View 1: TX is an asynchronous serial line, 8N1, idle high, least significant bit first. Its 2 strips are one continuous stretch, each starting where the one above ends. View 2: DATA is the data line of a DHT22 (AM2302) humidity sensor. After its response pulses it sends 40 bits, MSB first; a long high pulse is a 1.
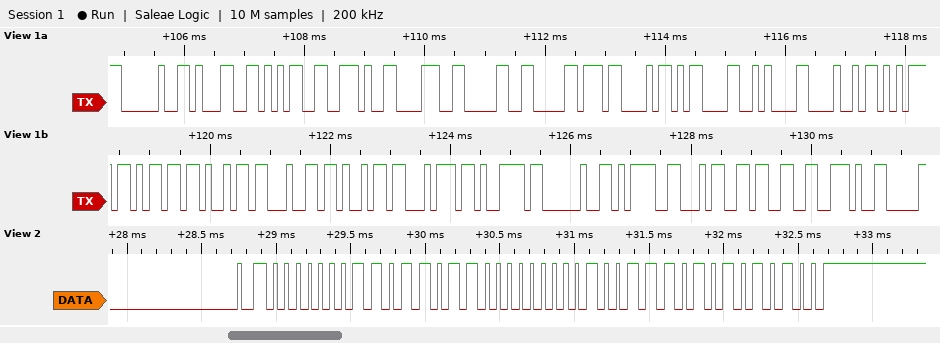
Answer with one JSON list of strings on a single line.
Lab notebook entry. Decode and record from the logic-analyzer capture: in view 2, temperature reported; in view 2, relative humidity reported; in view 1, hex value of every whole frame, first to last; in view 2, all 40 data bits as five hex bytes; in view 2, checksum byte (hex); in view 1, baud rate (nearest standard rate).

["15.7 °C", "43.8 %", "20 31 35 2E 38 30 B0 43 0D 0A 48 75 6D 69 64 69 74 79 20 3D 34 33 2E", "01 B6 00 9D 54", "0x54", "9600 baud"]
